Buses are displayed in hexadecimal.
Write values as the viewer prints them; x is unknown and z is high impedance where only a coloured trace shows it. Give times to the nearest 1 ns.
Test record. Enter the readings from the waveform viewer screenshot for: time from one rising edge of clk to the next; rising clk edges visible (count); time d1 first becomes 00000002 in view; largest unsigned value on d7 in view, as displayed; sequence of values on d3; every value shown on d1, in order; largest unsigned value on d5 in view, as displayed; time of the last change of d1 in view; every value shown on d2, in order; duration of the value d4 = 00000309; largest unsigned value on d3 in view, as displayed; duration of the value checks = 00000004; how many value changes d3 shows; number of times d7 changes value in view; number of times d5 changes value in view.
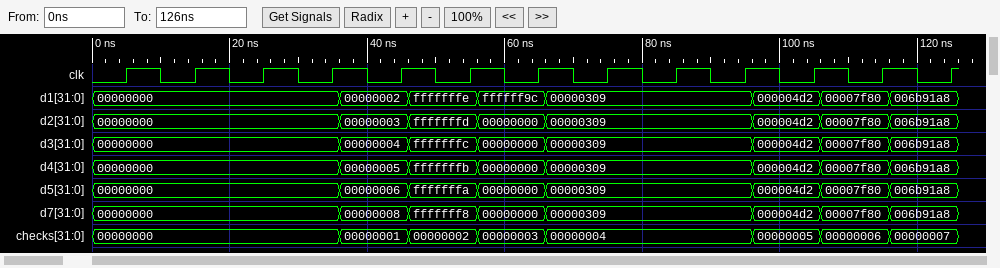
10 ns
13
36 ns
fffffff8
00000000, 00000004, fffffffc, 00000000, 00000309, 000004d2, 00007f80, 006b91a8
00000000, 00000002, fffffffe, ffffff9c, 00000309, 000004d2, 00007f80, 006b91a8
fffffffa
116 ns
00000000, 00000003, fffffffd, 00000000, 00000309, 000004d2, 00007f80, 006b91a8
30 ns
fffffffc
30 ns
7
7
7
